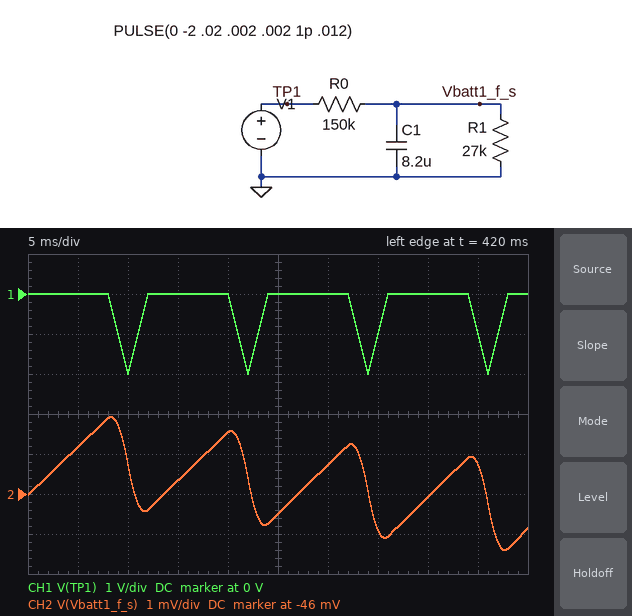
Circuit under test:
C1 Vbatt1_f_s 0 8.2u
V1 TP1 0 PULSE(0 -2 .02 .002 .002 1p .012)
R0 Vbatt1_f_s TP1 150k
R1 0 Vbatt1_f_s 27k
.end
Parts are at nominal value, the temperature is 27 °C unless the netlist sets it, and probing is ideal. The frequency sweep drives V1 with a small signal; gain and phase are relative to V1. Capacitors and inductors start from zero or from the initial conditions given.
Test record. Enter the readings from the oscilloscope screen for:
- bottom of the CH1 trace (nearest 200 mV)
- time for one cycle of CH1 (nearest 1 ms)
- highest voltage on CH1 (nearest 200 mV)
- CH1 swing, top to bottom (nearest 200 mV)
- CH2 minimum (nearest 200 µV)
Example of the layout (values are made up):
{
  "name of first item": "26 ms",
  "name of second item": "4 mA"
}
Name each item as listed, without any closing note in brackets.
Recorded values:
{
  "bottom of the CH1 trace": "-2.0 V",
  "time for one cycle of CH1": "12 ms",
  "highest voltage on CH1": "0 V",
  "CH1 swing, top to bottom": "2.0 V",
  "CH2 minimum": "-47.4 mV"
}
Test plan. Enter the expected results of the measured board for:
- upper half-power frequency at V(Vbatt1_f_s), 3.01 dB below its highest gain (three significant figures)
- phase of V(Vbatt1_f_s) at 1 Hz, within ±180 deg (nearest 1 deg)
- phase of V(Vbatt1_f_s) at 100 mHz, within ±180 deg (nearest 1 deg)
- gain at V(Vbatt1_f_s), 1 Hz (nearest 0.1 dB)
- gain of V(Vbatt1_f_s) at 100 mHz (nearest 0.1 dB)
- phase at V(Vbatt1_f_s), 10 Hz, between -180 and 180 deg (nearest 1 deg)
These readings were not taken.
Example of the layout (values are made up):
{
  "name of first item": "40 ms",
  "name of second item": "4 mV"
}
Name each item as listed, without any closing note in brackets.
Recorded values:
{
  "upper half-power frequency at V(Vbatt1_f_s), 3.01 dB below its highest gain": "848 mHz",
  "phase of V(Vbatt1_f_s) at 1 Hz, within ±180 deg": "-50 deg",
  "phase of V(Vbatt1_f_s) at 100 mHz, within ±180 deg": "-7 deg",
  "gain at V(Vbatt1_f_s), 1 Hz": "-20.1 dB",
  "gain of V(Vbatt1_f_s) at 100 mHz": "-16.4 dB",
  "phase at V(Vbatt1_f_s), 10 Hz, between -180 and 180 deg": "-85 deg"
}
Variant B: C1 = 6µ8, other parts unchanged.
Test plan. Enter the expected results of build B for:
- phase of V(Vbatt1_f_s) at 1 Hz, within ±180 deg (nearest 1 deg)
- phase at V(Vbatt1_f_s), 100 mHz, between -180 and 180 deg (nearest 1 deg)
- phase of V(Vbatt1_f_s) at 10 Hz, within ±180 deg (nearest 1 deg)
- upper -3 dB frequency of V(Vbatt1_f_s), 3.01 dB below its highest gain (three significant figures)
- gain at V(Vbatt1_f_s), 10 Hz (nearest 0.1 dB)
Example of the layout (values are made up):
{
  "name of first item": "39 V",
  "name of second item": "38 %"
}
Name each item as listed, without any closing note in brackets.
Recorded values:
{
  "phase of V(Vbatt1_f_s) at 1 Hz, within ±180 deg": "-44 deg",
  "phase at V(Vbatt1_f_s), 100 mHz, between -180 and 180 deg": "-6 deg",
  "phase of V(Vbatt1_f_s) at 10 Hz, within ±180 deg": "-84 deg",
  "upper -3 dB frequency of V(Vbatt1_f_s), 3.01 dB below its highest gain": "1.02 Hz",
  "gain at V(Vbatt1_f_s), 10 Hz": "-36.2 dB"
}
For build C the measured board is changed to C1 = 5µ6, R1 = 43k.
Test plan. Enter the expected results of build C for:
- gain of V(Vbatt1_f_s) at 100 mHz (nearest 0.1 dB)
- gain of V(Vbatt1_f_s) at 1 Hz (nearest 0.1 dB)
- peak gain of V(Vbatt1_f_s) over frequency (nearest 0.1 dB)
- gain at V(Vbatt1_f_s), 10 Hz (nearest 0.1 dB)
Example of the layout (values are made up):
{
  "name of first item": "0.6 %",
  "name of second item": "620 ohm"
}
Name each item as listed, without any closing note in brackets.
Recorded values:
{
  "gain of V(Vbatt1_f_s) at 100 mHz": "-13.1 dB",
  "gain of V(Vbatt1_f_s) at 1 Hz": "-16.8 dB",
  "peak gain of V(Vbatt1_f_s) over frequency": "-13.0 dB",
  "gain at V(Vbatt1_f_s), 10 Hz": "-34.5 dB"
}
